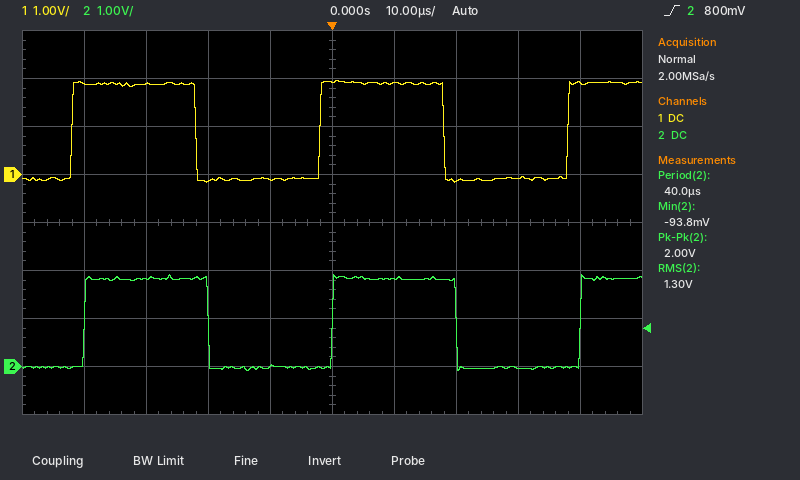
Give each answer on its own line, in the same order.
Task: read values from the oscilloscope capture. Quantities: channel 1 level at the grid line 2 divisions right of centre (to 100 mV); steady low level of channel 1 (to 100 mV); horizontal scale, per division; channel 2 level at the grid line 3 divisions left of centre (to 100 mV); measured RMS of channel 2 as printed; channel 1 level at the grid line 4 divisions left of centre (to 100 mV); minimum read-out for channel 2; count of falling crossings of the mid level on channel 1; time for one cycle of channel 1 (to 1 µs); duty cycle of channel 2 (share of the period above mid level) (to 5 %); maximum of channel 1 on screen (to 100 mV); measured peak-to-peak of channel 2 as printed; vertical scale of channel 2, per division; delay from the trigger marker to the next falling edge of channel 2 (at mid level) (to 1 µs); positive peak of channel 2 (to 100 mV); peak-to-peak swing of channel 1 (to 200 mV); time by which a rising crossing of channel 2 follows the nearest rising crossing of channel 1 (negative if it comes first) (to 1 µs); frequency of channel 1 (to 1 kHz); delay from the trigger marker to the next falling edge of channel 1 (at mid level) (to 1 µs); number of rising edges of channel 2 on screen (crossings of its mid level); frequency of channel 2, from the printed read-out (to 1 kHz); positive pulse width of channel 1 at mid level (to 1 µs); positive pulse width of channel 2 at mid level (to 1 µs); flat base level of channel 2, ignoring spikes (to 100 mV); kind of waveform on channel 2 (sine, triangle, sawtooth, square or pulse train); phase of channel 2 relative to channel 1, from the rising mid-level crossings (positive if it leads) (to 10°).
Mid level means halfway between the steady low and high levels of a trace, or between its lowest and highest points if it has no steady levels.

-100 mV
-100 mV
10 µs
1.8 V
1.30 V
1.9 V
-93.8 mV
2
40 µs
50 %
2.0 V
2.00 V
1 V
20 µs
1.9 V
2.2 V
+2 µs
25 kHz
18 µs
3
25 kHz
20 µs
20 µs
0.0 V
square
-20°
